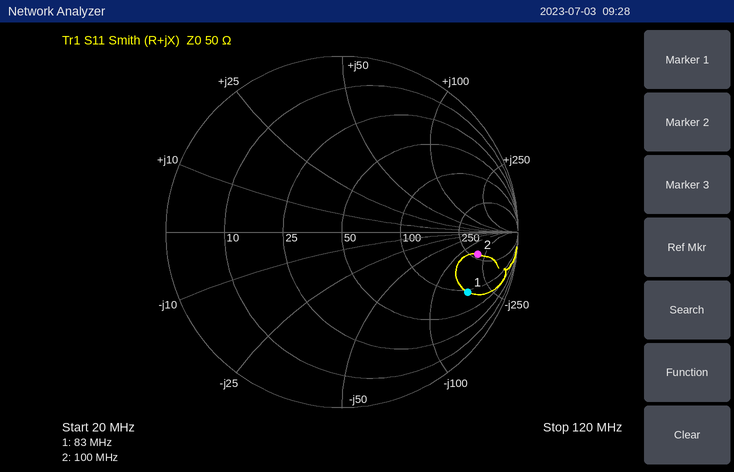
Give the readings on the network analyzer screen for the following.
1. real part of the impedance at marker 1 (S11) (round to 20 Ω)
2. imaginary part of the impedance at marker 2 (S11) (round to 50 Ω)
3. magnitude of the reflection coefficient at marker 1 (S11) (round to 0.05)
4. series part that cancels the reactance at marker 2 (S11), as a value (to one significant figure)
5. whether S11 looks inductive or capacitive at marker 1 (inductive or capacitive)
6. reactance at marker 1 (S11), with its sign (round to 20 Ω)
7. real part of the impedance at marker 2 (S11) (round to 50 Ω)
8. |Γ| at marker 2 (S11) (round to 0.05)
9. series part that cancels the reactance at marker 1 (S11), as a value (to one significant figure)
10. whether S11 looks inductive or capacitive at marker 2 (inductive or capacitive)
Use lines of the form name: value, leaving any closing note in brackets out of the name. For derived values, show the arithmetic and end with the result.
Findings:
real part of the impedance at marker 1 (S11): 100 Ω
imaginary part of the impedance at marker 2 (S11): -200 Ω
magnitude of the reflection coefficient at marker 1 (S11): 0.80
series part that cancels the reactance at marker 2 (S11), as a value: L = 200 Ω/(2π × 100 MHz) ≈ 318 nH, so 300 nH to one significant figure
whether S11 looks inductive or capacitive at marker 1: capacitive
reactance at marker 1 (S11), with its sign: -180 Ω
real part of the impedance at marker 2 (S11): 300 Ω
|Γ| at marker 2 (S11): 0.80
series part that cancels the reactance at marker 1 (S11), as a value: L = 180 Ω/(2π × 83 MHz) ≈ 345 nH, so 300 nH to one significant figure
whether S11 looks inductive or capacitive at marker 2: capacitive
